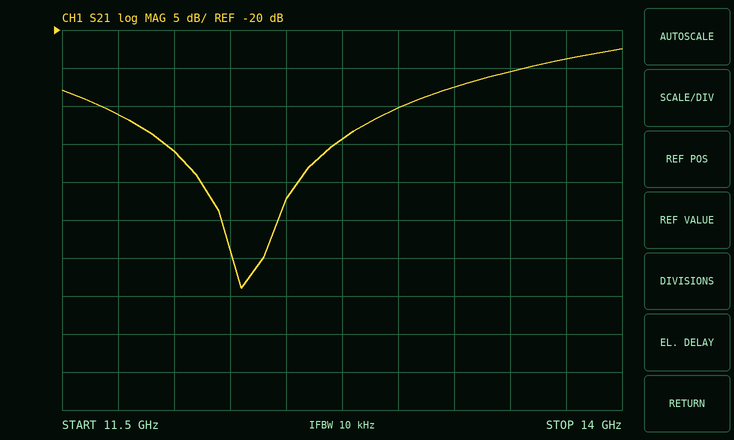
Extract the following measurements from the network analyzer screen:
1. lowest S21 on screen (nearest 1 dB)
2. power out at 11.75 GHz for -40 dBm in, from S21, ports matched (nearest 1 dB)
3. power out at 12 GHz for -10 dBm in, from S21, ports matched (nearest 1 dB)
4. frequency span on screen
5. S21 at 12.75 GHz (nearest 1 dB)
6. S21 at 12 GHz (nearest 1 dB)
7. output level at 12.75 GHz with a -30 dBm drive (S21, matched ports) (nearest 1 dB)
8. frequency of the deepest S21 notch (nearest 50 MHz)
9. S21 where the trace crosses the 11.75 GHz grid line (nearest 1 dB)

-54 dB
-71 dBm
-46 dBm
2.5 GHz
-34 dB
-36 dB
-64 dBm
12.30 GHz
-31 dB
